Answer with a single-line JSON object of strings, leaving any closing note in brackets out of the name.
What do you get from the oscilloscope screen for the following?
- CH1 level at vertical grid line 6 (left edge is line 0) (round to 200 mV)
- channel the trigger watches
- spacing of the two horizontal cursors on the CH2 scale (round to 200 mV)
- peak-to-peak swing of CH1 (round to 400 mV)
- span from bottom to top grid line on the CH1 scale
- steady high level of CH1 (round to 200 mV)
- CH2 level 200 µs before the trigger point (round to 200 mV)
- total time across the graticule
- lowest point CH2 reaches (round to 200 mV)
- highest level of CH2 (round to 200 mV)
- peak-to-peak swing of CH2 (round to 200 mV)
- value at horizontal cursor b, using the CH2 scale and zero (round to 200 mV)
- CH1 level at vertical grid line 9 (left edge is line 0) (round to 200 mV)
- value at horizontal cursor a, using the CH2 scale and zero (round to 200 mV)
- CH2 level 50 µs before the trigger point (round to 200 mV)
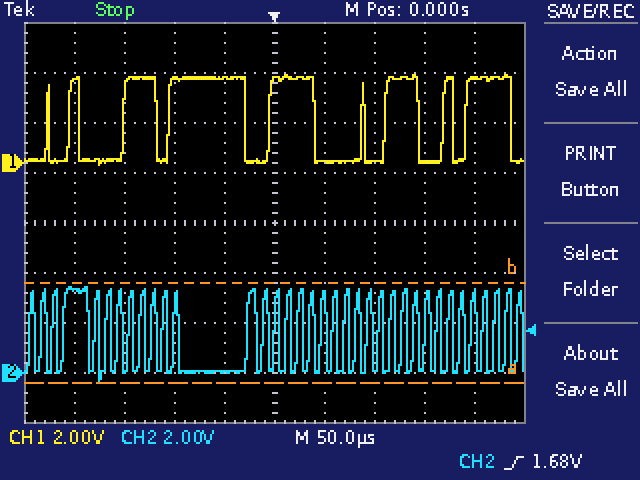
{"CH1 level at vertical grid line 6 (left edge is line 0)": "0.0 V", "channel the trigger watches": "CH2", "spacing of the two horizontal cursors on the CH2 scale": "4.0 V", "peak-to-peak swing of CH1": "3.6 V", "span from bottom to top grid line on the CH1 scale": "16 V", "steady high level of CH1": "3.4 V", "CH2 level 200 µs before the trigger point": "3.4 V", "total time across the graticule": "500 µs", "lowest point CH2 reaches": "-400 mV", "highest level of CH2": "3.4 V", "peak-to-peak swing of CH2": "3.8 V", "value at horizontal cursor b, using the CH2 scale and zero": "3.6 V", "CH1 level at vertical grid line 9 (left edge is line 0)": "3.4 V", "value at horizontal cursor a, using the CH2 scale and zero": "-400 mV", "CH2 level 50 µs before the trigger point": "0.0 V"}
